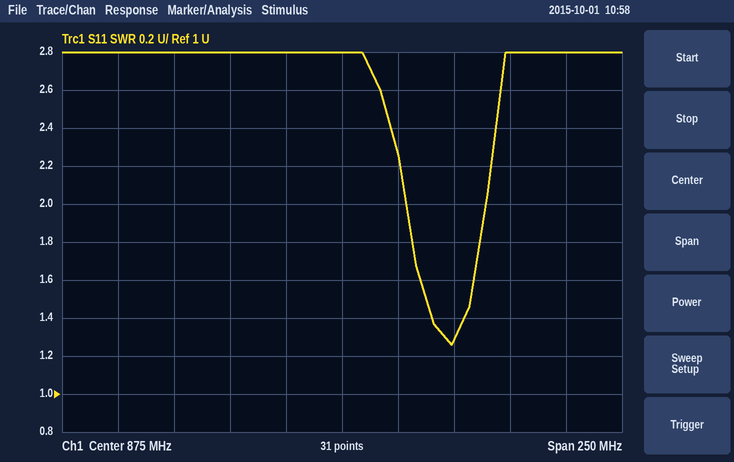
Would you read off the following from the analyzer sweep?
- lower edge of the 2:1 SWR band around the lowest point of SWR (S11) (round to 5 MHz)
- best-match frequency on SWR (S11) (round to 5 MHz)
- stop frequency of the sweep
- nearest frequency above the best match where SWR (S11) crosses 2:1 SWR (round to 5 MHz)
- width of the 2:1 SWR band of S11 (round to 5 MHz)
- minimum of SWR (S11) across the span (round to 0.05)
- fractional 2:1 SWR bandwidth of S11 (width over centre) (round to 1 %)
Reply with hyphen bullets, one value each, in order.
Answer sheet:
- 905 MHz
- 925 MHz
- 1 GHz
- 940 MHz
- 35 MHz
- 1.25
- 4 %
